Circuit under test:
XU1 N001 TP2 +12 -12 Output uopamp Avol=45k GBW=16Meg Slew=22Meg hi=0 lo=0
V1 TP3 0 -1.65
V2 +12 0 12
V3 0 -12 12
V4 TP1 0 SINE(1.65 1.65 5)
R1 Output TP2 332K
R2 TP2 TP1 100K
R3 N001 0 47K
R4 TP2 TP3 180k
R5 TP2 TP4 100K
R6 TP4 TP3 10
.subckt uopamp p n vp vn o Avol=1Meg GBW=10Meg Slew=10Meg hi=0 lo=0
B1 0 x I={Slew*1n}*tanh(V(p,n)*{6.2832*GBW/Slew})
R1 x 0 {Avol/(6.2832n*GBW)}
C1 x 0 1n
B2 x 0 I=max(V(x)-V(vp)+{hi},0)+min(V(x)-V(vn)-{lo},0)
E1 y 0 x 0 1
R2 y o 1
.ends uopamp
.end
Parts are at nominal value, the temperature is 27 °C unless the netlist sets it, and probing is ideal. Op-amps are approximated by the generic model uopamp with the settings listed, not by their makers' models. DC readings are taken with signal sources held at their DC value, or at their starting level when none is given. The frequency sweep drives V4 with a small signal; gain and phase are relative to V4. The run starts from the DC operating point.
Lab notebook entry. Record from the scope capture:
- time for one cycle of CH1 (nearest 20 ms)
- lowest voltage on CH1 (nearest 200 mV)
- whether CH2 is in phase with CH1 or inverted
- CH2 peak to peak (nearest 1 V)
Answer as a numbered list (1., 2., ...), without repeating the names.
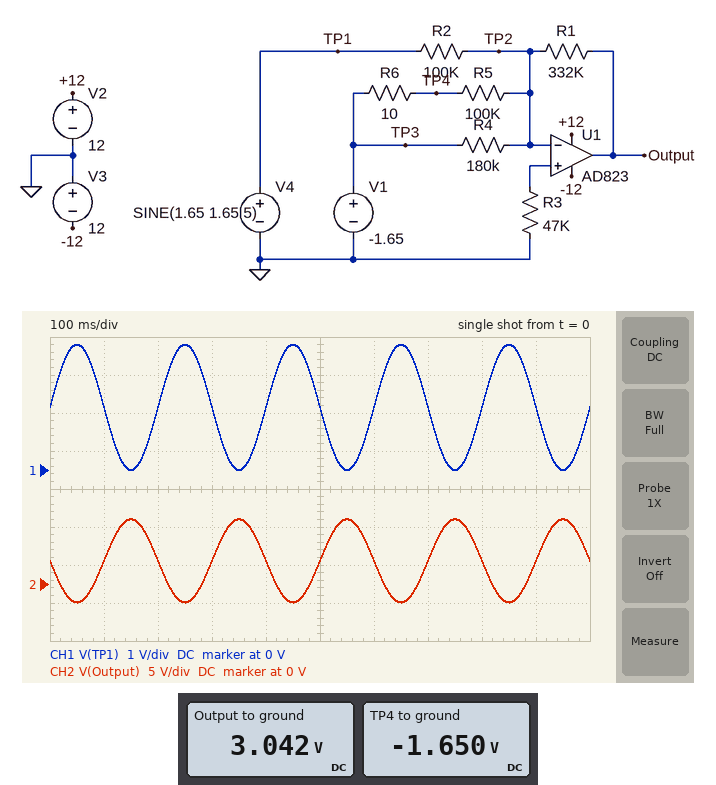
1. 200 ms
2. 0 V
3. inverted
4. 11 V
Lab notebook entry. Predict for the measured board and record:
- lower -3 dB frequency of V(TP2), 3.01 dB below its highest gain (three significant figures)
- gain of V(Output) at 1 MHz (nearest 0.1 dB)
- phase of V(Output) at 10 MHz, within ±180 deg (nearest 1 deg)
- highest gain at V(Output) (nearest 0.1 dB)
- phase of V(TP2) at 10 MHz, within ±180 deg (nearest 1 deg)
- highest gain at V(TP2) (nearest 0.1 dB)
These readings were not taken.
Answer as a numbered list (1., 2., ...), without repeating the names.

1. 1.69 MHz
2. 9.1 dB
3. 100 deg
4. 10.4 dB
5. 10 deg
6. -9.1 dB
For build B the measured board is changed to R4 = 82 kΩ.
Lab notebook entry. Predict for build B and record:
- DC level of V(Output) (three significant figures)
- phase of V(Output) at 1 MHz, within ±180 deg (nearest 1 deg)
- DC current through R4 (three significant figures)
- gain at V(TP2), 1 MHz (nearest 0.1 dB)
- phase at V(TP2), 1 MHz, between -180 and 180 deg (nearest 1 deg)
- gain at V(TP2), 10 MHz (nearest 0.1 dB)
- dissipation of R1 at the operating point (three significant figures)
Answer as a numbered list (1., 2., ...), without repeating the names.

1. 6.68 V
2. 144 deg
3. 20.1 µA
4. -15.5 dB
5. 54 deg
6. -11.0 dB
7. 134 µW
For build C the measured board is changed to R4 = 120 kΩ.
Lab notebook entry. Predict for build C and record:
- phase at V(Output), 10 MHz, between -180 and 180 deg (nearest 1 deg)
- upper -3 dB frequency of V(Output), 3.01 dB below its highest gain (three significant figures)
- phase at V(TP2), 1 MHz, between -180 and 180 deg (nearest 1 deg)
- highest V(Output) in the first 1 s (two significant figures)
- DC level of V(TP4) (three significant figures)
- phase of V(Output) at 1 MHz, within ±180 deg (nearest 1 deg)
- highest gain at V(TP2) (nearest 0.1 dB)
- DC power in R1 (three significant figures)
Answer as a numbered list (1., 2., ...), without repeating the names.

1. 99 deg
2. 1.54 MHz
3. 57 deg
4. 10 V
5. -1.65 V
6. 147 deg
7. -9.9 dB
8. 62.7 µW
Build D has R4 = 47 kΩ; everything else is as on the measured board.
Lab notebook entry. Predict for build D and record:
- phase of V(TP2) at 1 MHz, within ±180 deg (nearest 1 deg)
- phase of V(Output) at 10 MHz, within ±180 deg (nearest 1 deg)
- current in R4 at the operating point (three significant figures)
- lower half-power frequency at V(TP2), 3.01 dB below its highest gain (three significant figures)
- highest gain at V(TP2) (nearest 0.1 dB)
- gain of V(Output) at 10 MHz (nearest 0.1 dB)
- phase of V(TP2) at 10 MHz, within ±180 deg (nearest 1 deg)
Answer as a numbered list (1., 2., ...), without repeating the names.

1. 47 deg
2. 96 deg
3. 35.1 µA
4. 1.09 MHz
5. -12.9 dB
6. -8.9 dB
7. 6 deg
